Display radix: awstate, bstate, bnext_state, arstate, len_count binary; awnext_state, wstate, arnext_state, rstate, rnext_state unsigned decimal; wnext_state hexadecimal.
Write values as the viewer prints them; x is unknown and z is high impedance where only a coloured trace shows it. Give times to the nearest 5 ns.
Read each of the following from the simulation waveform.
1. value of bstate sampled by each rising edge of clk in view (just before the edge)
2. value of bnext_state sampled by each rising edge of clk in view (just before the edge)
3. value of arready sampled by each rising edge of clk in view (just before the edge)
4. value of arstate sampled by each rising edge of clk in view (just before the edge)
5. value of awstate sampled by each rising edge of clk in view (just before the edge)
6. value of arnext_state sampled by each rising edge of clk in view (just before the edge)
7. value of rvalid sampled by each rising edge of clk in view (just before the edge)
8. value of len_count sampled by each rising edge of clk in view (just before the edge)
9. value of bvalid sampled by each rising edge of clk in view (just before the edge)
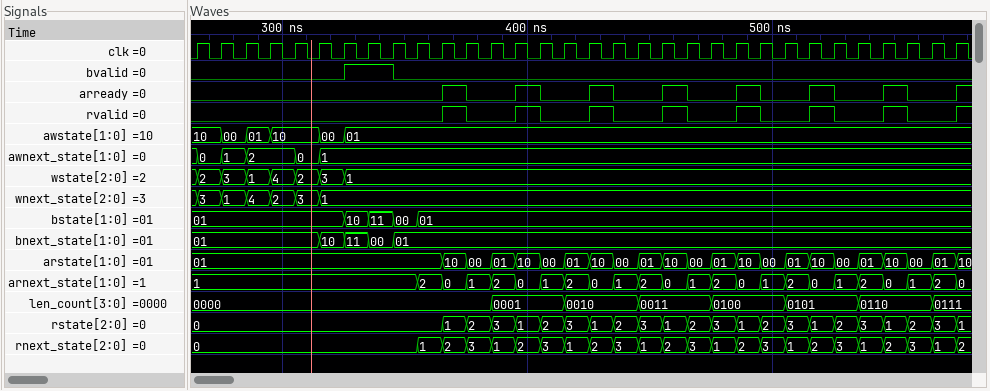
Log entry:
01, 01, 01, 01, 01, 01, 01, 10, 11, 00, 01, 01, 01, 01, 01, 01, 01, 01, 01, 01, 01, 01, 01, 01, 01, 01, 01, 01, 01, 01, 01, 01
01, 01, 01, 01, 01, 01, 10, 11, 00, 01, 01, 01, 01, 01, 01, 01, 01, 01, 01, 01, 01, 01, 01, 01, 01, 01, 01, 01, 01, 01, 01, 01
0 0 0 0 0 0 0 0 0 0 0 1 0 0 1 0 0 1 0 0 1 0 0 1 0 0 1 0 0 1 0 0
01, 01, 01, 01, 01, 01, 01, 01, 01, 01, 01, 10, 00, 01, 10, 00, 01, 10, 00, 01, 10, 00, 01, 10, 00, 01, 10, 00, 01, 10, 00, 01
10, 10, 00, 01, 10, 10, 00, 01, 01, 01, 01, 01, 01, 01, 01, 01, 01, 01, 01, 01, 01, 01, 01, 01, 01, 01, 01, 01, 01, 01, 01, 01
1, 1, 1, 1, 1, 1, 1, 1, 1, 1, 2, 0, 1, 2, 0, 1, 2, 0, 1, 2, 0, 1, 2, 0, 1, 2, 0, 1, 2, 0, 1, 2
0 0 0 0 0 0 0 0 0 0 0 1 0 0 1 0 0 1 0 0 1 0 0 1 0 0 1 0 0 1 0 0
0000, 0000, 0000, 0000, 0000, 0000, 0000, 0000, 0000, 0000, 0000, 0000, 0000, 0001, 0001, 0001, 0010, 0010, 0010, 0011, 0011, 0011, 0100, 0100, 0100, 0101, 0101, 0101, 0110, 0110, 0110, 0111
0 0 0 0 0 0 0 1 1 0 0 0 0 0 0 0 0 0 0 0 0 0 0 0 0 0 0 0 0 0 0 0
